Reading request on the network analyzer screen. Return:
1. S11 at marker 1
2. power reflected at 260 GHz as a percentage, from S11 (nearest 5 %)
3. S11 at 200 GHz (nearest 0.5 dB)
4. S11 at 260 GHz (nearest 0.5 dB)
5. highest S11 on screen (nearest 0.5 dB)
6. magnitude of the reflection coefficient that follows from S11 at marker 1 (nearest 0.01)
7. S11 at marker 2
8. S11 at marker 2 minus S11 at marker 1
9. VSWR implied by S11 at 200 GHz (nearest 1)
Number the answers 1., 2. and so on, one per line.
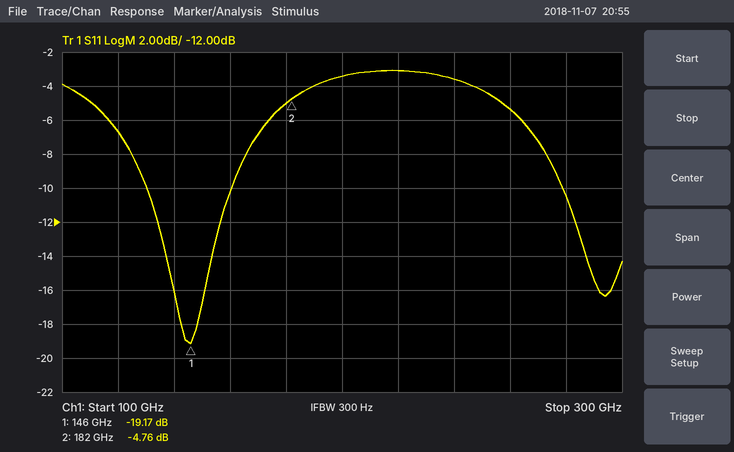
1. -19.17 dB
2. 30 %
3. -3.5 dB
4. -5.5 dB
5. -3.0 dB
6. 0.11
7. -4.76 dB
8. 14.41 dB
9. 5
